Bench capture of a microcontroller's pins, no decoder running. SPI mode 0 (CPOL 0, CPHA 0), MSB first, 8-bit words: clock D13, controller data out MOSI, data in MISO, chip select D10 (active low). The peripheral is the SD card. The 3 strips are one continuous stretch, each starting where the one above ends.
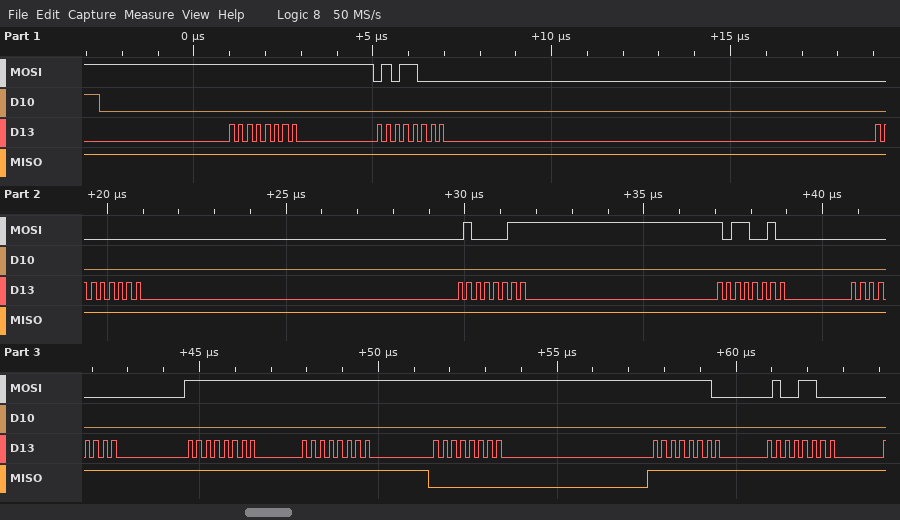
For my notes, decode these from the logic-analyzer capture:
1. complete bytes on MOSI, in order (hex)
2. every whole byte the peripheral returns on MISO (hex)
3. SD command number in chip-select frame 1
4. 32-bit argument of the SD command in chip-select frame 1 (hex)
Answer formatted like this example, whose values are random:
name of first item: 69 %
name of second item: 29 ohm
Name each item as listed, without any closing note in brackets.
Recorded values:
complete bytes on MOSI, in order: 0xFF 0x58 0x00 0x43 0xB2 0x00 0xFF 0xFF 0xFF 0xFE 0x4C
every whole byte the peripheral returns on MISO: 0xFF 0xFF 0xFF 0xFF 0xFF 0xFF 0xFF 0xFF 0x00 0xFF 0xFF
SD command number in chip-select frame 1: CMD24
32-bit argument of the SD command in chip-select frame 1: 0x0043B200
